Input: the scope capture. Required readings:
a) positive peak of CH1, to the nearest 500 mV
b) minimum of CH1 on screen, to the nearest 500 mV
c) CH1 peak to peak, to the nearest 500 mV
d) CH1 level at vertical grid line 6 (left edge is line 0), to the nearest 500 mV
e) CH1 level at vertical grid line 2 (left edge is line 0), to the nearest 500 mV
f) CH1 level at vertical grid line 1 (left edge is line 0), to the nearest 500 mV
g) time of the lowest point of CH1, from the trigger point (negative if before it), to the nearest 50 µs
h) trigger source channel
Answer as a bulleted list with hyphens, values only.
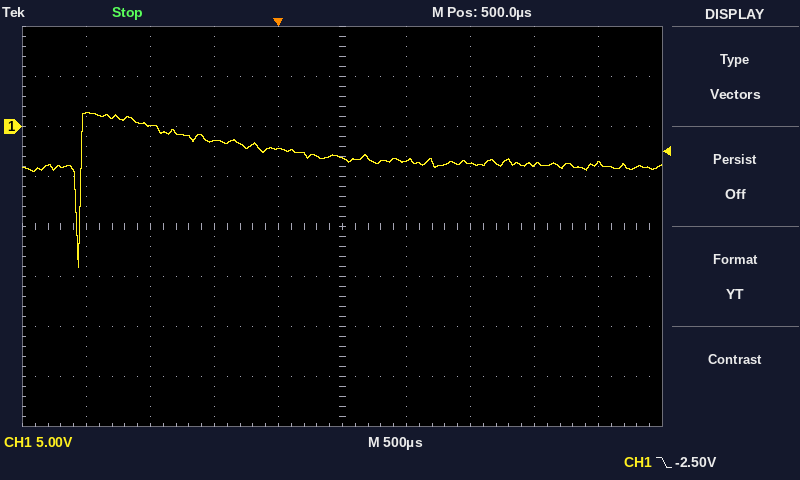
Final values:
- 1.5 V
- -14.0 V
- 15.5 V
- -3.5 V
- 0.0 V
- 1.5 V
- -1.55 ms
- CH1
